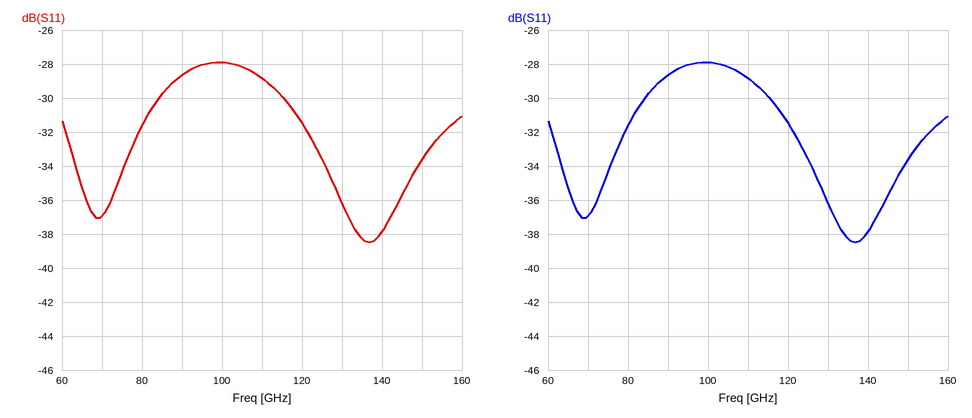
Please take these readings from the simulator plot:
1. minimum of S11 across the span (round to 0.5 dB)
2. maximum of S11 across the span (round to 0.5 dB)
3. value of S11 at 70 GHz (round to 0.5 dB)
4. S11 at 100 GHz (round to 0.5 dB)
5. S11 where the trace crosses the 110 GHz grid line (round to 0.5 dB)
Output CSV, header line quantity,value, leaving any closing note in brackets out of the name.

quantity,value
minimum of S11 across the span,-38.5 dB
maximum of S11 across the span,-28.0 dB
value of S11 at 70 GHz,-37.0 dB
S11 at 100 GHz,-28.0 dB
S11 where the trace crosses the 110 GHz grid line,-29.0 dB
